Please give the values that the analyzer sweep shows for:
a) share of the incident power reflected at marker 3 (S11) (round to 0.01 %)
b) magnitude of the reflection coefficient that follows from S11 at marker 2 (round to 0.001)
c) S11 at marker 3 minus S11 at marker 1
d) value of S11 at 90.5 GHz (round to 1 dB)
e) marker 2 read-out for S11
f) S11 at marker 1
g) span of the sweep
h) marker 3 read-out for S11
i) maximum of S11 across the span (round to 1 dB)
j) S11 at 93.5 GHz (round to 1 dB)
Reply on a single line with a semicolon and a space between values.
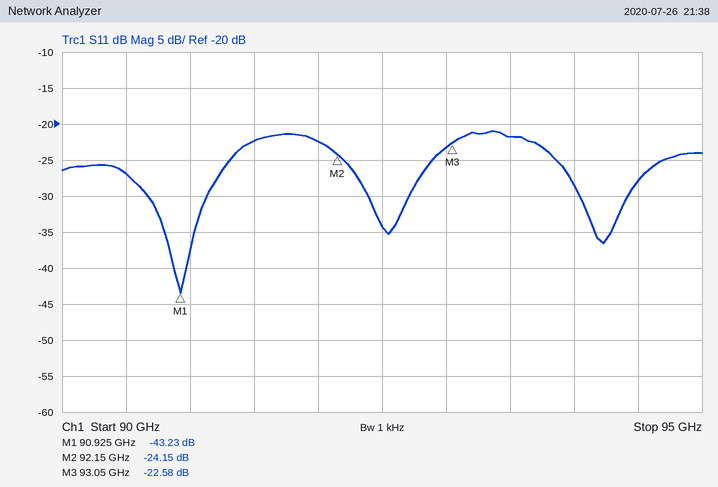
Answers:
0.55 %; 0.062; 20.65 dB; -27 dB; -24.15 dB; -43.23 dB; 5 GHz; -22.58 dB; -21 dB; -22 dB
